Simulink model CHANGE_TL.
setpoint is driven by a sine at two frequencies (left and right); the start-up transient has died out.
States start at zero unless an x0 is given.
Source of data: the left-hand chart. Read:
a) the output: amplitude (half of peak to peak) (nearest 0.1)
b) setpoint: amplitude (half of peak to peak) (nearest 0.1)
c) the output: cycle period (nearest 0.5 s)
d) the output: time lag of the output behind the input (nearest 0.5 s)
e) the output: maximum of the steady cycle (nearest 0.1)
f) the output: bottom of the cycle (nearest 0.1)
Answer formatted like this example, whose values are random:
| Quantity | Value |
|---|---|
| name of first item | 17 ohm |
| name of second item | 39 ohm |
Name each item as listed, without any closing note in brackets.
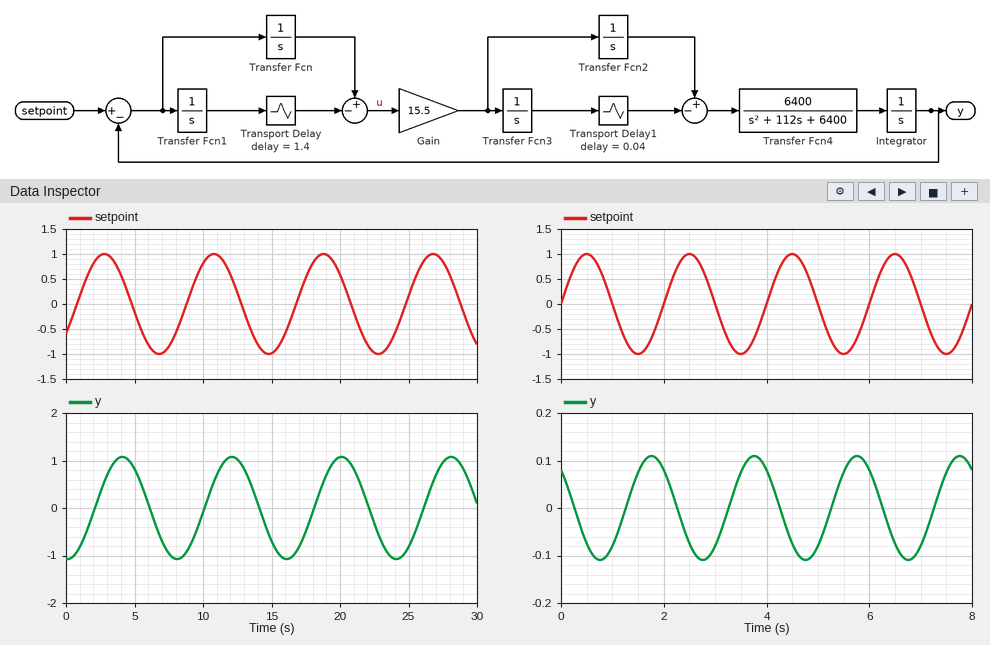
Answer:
| Quantity | Value |
|---|---|
| the output: amplitude (half of peak to peak) | 1.1 |
| setpoint: amplitude (half of peak to peak) | 1.0 |
| the output: cycle period | 8.0 s |
| the output: time lag of the output behind the input | 1.5 s |
| the output: maximum of the steady cycle | 1.1 |
| the output: bottom of the cycle | -1.1 |
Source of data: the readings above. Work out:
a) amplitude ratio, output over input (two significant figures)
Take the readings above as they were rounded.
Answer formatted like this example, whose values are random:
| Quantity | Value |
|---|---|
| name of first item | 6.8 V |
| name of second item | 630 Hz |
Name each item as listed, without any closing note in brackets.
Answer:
| Quantity | Value |
|---|---|
| amplitude ratio, output over input | 1.1 |
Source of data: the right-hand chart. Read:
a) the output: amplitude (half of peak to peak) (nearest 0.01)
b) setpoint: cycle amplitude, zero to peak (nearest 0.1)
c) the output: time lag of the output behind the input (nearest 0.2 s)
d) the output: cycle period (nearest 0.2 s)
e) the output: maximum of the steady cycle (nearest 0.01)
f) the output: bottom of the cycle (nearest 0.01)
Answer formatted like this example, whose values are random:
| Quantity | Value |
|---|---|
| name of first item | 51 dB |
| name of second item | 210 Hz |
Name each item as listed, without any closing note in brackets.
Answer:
| Quantity | Value |
|---|---|
| the output: amplitude (half of peak to peak) | 0.11 |
| setpoint: cycle amplitude, zero to peak | 1.0 |
| the output: time lag of the output behind the input | 1.2 s |
| the output: cycle period | 2.0 s |
| the output: maximum of the steady cycle | 0.11 |
| the output: bottom of the cycle | -0.11 |
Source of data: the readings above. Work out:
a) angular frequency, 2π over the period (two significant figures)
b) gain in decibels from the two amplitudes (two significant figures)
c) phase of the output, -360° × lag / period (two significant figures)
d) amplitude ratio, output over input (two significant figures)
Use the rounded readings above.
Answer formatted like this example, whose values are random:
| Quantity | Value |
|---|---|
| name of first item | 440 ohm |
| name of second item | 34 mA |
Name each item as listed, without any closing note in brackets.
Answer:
| Quantity | Value |
|---|---|
| angular frequency, 2π over the period | 3.1 rad/s |
| gain in decibels from the two amplitudes | -19 dB |
| phase of the output, -360° × lag / period | -220° |
| amplitude ratio, output over input | 0.11 |
